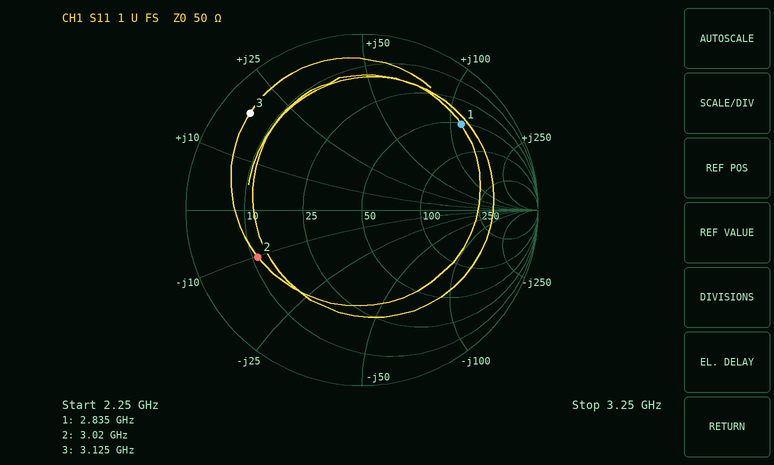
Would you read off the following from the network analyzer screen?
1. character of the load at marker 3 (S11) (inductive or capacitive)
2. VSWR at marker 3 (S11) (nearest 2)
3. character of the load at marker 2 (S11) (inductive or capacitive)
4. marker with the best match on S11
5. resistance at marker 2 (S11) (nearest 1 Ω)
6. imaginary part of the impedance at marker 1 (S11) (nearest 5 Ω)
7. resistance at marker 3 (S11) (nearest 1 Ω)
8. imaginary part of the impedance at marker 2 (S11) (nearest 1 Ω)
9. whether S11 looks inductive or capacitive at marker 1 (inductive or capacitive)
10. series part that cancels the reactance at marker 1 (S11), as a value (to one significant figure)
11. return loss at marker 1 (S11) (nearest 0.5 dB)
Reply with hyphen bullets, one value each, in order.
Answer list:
- inductive
- 12
- capacitive
- marker 2
- 11 Ω
- +115 Ω
- 5 Ω
- -10 Ω
- inductive
- 500 fF
- 2.5 dB
